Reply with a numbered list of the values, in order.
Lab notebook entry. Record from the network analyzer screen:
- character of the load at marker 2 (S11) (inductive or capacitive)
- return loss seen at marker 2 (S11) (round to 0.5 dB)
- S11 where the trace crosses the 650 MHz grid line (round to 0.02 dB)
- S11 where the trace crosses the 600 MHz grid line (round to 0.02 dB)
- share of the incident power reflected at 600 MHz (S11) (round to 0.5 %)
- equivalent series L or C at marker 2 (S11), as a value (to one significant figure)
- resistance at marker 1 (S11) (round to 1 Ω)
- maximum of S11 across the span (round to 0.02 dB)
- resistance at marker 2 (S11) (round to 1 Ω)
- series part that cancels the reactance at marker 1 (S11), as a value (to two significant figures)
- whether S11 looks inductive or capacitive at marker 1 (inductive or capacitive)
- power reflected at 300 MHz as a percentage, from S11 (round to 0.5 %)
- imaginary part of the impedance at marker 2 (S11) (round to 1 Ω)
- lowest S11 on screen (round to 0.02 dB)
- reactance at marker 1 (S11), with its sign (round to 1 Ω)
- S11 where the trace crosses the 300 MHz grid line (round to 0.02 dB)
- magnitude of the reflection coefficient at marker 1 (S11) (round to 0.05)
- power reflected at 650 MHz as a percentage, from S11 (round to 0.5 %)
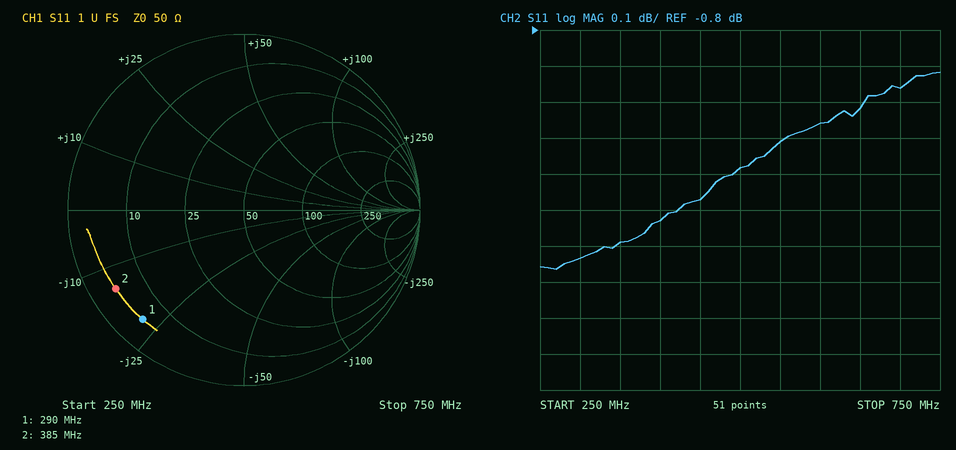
1. capacitive
2. 1.5 dB
3. -1.02 dB
4. -1.06 dB
5. 78.5 %
6. 30 pF
7. 5 Ω
8. -0.92 dB
9. 4 Ω
10. 12 nH
11. capacitive
12. 72.0 %
13. -14 Ω
14. -1.46 dB
15. -22 Ω
16. -1.44 dB
17. 0.85
18. 79.0 %
